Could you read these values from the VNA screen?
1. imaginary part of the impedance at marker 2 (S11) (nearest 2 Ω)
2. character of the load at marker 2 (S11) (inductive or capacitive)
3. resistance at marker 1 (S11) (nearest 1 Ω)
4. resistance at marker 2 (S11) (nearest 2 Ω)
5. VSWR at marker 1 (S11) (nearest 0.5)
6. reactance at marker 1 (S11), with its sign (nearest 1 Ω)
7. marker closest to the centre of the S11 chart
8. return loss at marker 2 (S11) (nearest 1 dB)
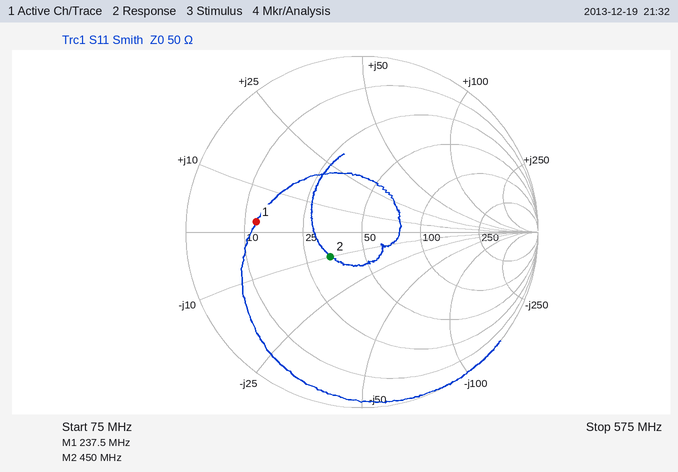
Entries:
-10 Ω
capacitive
12 Ω
34 Ω
4.0
+2 Ω
marker 2
13 dB
